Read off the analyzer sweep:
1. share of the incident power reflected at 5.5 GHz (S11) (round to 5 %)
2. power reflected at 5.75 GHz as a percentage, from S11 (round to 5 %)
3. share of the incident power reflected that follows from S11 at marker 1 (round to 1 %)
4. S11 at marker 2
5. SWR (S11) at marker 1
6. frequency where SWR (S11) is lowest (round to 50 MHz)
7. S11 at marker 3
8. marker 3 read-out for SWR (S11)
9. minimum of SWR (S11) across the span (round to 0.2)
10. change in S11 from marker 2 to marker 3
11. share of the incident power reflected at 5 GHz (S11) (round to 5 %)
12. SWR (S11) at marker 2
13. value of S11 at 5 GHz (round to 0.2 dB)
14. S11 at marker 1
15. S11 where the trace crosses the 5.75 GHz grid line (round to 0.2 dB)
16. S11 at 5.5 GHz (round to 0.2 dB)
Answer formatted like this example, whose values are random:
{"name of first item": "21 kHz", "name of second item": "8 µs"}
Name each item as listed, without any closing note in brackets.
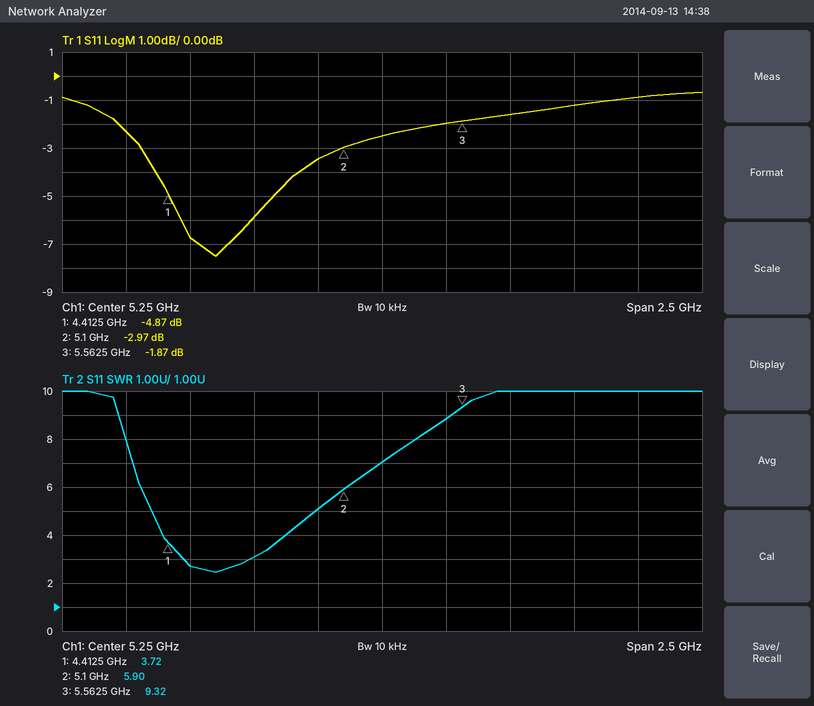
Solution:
{"share of the incident power reflected at 5.5 GHz (S11)": "65 %", "power reflected at 5.75 GHz as a percentage, from S11": "70 %", "share of the incident power reflected that follows from S11 at marker 1": "33 %", "S11 at marker 2": "-2.97 dB", "SWR (S11) at marker 1": "3.72", "frequency where SWR (S11) is lowest": "4.60 GHz", "S11 at marker 3": "-1.87 dB", "marker 3 read-out for SWR": "9.32", "minimum of SWR (S11) across the span": "2.4", "change in S11 from marker 2 to marker 3": "1.10 dB", "share of the incident power reflected at 5 GHz (S11)": "45 %", "SWR (S11) at marker 2": "5.90", "value of S11 at 5 GHz": "-3.4 dB", "S11 at marker 1": "-4.87 dB", "S11 where the trace crosses the 5.75 GHz grid line": "-1.6 dB", "S11 at 5.5 GHz": "-2.0 dB"}
